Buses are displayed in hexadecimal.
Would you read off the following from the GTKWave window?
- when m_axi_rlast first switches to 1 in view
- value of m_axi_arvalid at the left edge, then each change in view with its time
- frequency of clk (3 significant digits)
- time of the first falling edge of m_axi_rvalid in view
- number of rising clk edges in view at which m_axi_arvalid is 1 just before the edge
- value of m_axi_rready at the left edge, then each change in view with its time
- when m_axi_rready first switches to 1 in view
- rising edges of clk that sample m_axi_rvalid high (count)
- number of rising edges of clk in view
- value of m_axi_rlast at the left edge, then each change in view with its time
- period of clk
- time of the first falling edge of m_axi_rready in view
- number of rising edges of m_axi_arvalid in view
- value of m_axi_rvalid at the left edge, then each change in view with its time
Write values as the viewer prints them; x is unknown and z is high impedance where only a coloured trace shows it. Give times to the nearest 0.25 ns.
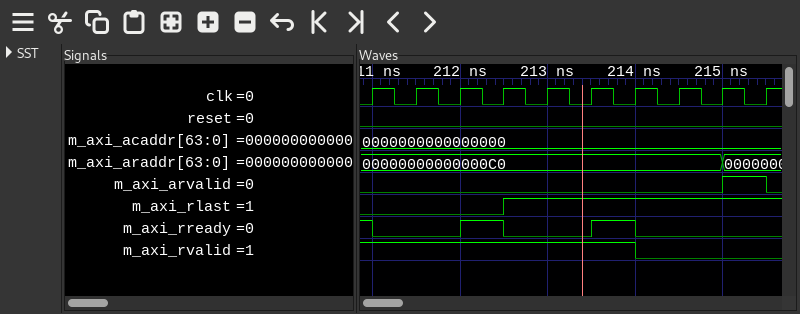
212.5 ns
0, 1 at 215 ns, 0 at 215.5 ns
2.00 GHz
214 ns
1
1, 0 at 211 ns, 1 at 212 ns, 0 at 212.5 ns, 1 at 213.5 ns, 0 at 214 ns
212 ns
7
10
0, 1 at 212.5 ns
0.5 ns
211 ns
1
1, 0 at 214 ns
